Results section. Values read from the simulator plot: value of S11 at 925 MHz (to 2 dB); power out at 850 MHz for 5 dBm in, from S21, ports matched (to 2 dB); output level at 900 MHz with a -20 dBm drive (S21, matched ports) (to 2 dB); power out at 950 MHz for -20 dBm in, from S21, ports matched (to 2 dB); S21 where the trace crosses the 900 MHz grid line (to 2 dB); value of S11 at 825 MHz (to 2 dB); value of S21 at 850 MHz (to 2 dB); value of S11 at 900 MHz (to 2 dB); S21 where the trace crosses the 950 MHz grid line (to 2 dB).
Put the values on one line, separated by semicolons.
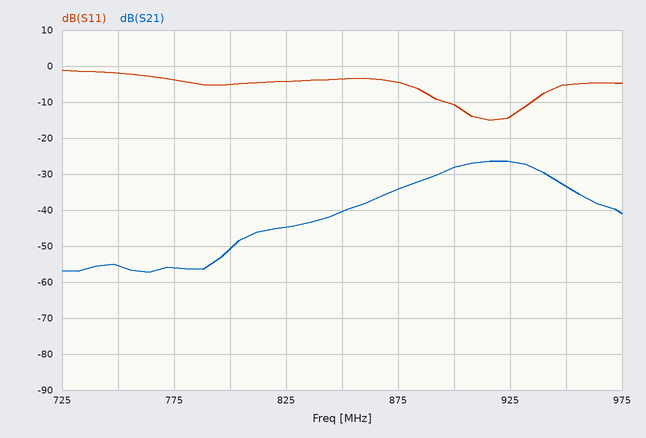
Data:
-14 dB; -36 dBm; -48 dBm; -54 dBm; -28 dB; -4 dB; -40 dB; -10 dB; -34 dB
